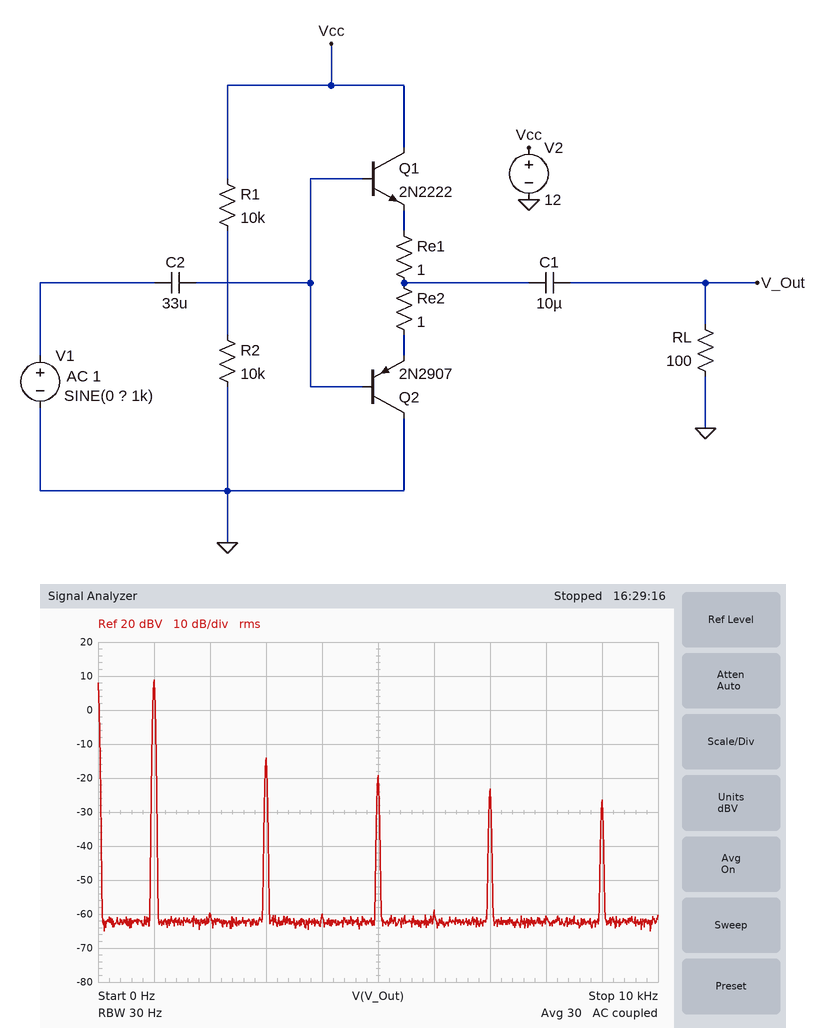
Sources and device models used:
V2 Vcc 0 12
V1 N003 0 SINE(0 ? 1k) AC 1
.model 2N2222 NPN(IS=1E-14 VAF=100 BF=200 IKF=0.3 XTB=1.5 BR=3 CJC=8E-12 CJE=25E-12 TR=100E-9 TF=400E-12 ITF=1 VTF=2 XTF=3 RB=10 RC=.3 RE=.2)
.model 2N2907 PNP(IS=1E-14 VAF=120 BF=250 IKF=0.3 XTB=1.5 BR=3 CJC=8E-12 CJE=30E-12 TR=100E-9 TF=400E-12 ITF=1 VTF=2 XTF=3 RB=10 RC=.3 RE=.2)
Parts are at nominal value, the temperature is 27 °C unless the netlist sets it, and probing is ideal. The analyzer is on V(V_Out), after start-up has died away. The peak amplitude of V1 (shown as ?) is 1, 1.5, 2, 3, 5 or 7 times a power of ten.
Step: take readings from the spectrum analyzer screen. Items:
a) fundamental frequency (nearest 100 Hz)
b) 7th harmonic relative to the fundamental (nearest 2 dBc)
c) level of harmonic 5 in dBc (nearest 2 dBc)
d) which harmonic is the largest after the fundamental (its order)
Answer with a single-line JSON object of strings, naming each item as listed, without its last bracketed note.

{"fundamental frequency": "1.0 kHz", "7th harmonic relative to the fundamental": "-32 dBc", "level of harmonic 5 in dBc": "-28 dBc", "which harmonic is the largest after the fundamental": "3"}
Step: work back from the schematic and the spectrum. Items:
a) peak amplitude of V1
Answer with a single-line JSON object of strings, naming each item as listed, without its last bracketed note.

{"peak amplitude of V1": "5 V"}
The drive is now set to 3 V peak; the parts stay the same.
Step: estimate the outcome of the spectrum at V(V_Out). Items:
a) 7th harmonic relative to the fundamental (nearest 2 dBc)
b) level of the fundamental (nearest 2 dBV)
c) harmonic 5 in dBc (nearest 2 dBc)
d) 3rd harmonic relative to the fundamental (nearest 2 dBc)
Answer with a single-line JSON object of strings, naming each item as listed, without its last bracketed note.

{"7th harmonic relative to the fundamental": "-30 dBc", "level of the fundamental": "4 dBV", "harmonic 5 in dBc": "-24 dBc", "3rd harmonic relative to the fundamental": "-18 dBc"}
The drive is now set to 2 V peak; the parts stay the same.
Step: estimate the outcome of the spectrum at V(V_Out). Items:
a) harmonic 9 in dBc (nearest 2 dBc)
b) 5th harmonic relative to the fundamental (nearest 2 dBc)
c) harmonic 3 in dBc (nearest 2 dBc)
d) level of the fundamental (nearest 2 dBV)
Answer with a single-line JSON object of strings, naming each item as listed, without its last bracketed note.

{"harmonic 9 in dBc": "-48 dBc", "5th harmonic relative to the fundamental": "-22 dBc", "harmonic 3 in dBc": "-14 dBc", "level of the fundamental": "-2 dBV"}
